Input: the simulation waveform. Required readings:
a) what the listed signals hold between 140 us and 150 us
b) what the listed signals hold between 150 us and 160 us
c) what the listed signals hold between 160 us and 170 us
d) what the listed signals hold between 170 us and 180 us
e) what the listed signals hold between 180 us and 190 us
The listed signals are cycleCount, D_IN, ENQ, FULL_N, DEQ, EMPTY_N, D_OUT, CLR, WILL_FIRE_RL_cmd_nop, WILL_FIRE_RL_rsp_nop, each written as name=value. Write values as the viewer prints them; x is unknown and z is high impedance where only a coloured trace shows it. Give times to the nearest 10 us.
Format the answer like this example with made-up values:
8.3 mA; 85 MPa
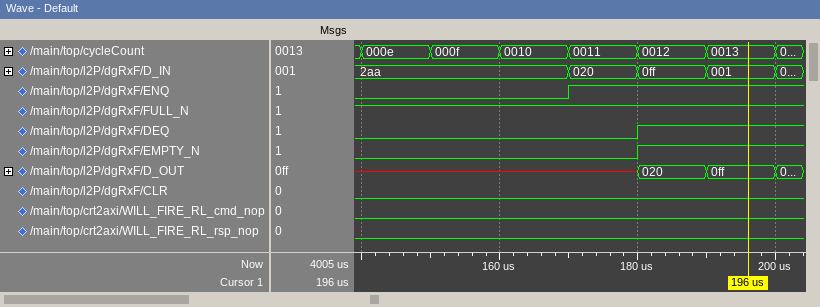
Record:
cycleCount=000e, D_IN=2aa, ENQ=0, FULL_N=1, DEQ=0, EMPTY_N=0, D_OUT=x, CLR=0, WILL_FIRE_RL_cmd_nop=0, WILL_FIRE_RL_rsp_nop=0; cycleCount=000f, D_IN=2aa, ENQ=0, FULL_N=1, DEQ=0, EMPTY_N=0, D_OUT=x, CLR=0, WILL_FIRE_RL_cmd_nop=0, WILL_FIRE_RL_rsp_nop=0; cycleCount=0010, D_IN=2aa, ENQ=0, FULL_N=1, DEQ=0, EMPTY_N=0, D_OUT=x, CLR=0, WILL_FIRE_RL_cmd_nop=0, WILL_FIRE_RL_rsp_nop=0; cycleCount=0011, D_IN=020, ENQ=1, FULL_N=1, DEQ=0, EMPTY_N=0, D_OUT=x, CLR=0, WILL_FIRE_RL_cmd_nop=0, WILL_FIRE_RL_rsp_nop=0; cycleCount=0012, D_IN=0ff, ENQ=1, FULL_N=1, DEQ=1, EMPTY_N=1, D_OUT=020, CLR=0, WILL_FIRE_RL_cmd_nop=0, WILL_FIRE_RL_rsp_nop=0
